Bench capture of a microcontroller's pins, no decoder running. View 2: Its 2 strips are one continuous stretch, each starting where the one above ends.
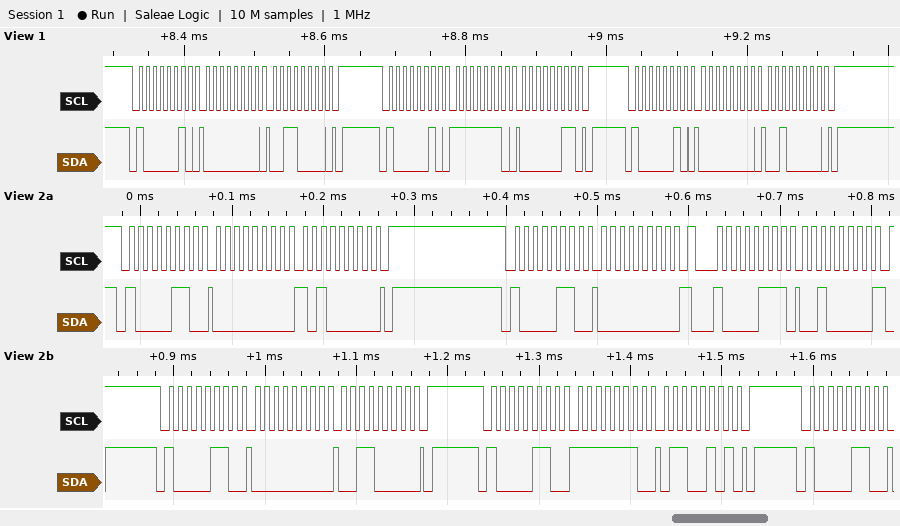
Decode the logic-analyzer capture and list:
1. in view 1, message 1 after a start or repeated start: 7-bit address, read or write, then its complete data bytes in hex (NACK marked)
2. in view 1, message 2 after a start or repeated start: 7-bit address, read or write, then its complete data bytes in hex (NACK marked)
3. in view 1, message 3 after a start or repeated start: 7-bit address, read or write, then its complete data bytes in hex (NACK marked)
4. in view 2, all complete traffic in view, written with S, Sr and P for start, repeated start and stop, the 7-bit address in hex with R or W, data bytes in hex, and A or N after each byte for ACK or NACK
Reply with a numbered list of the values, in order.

1. 0x41 write: 00 30
2. 0x41 write: FE 03
3. 0x41 write: 00 20
4. S 43W A 00 A A0 A P S 43W A 00 A Sr 43R A 20 N P S 43W A 00 A 30 A P S 43W A FE A 65 A P S 43W A
